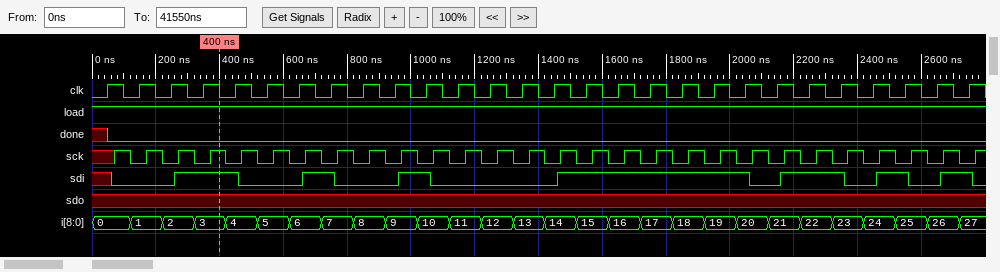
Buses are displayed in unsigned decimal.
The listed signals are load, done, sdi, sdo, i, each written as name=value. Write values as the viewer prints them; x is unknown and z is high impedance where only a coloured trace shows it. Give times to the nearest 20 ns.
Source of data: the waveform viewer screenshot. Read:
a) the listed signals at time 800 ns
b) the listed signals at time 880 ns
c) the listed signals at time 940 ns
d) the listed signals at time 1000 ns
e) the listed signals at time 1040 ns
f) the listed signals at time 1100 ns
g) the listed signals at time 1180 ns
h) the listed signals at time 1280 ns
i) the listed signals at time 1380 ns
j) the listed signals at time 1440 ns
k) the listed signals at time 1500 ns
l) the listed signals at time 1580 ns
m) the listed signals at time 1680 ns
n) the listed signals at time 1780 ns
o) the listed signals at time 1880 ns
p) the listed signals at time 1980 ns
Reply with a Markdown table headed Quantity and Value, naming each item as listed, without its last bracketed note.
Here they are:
| Quantity | Value |
|---|---|
| the listed signals at time 800 ns | load=1, done=0, sdi=0, sdo=x, i=7 |
| the listed signals at time 880 ns | load=1, done=0, sdi=0, sdo=x, i=8 |
| the listed signals at time 940 ns | load=1, done=0, sdi=0, sdo=x, i=9 |
| the listed signals at time 1000 ns | load=1, done=0, sdi=1, sdo=x, i=9 |
| the listed signals at time 1040 ns | load=1, done=0, sdi=1, sdo=x, i=10 |
| the listed signals at time 1100 ns | load=1, done=0, sdi=0, sdo=x, i=10 |
| the listed signals at time 1180 ns | load=1, done=0, sdi=0, sdo=x, i=11 |
| the listed signals at time 1280 ns | load=1, done=0, sdi=0, sdo=x, i=12 |
| the listed signals at time 1380 ns | load=1, done=0, sdi=0, sdo=x, i=13 |
| the listed signals at time 1440 ns | load=1, done=0, sdi=0, sdo=x, i=14 |
| the listed signals at time 1500 ns | load=1, done=0, sdi=1, sdo=x, i=14 |
| the listed signals at time 1580 ns | load=1, done=0, sdi=1, sdo=x, i=15 |
| the listed signals at time 1680 ns | load=1, done=0, sdi=1, sdo=x, i=16 |
| the listed signals at time 1780 ns | load=1, done=0, sdi=1, sdo=x, i=17 |
| the listed signals at time 1880 ns | load=1, done=0, sdi=1, sdo=x, i=18 |
| the listed signals at time 1980 ns | load=1, done=0, sdi=1, sdo=x, i=19 |
